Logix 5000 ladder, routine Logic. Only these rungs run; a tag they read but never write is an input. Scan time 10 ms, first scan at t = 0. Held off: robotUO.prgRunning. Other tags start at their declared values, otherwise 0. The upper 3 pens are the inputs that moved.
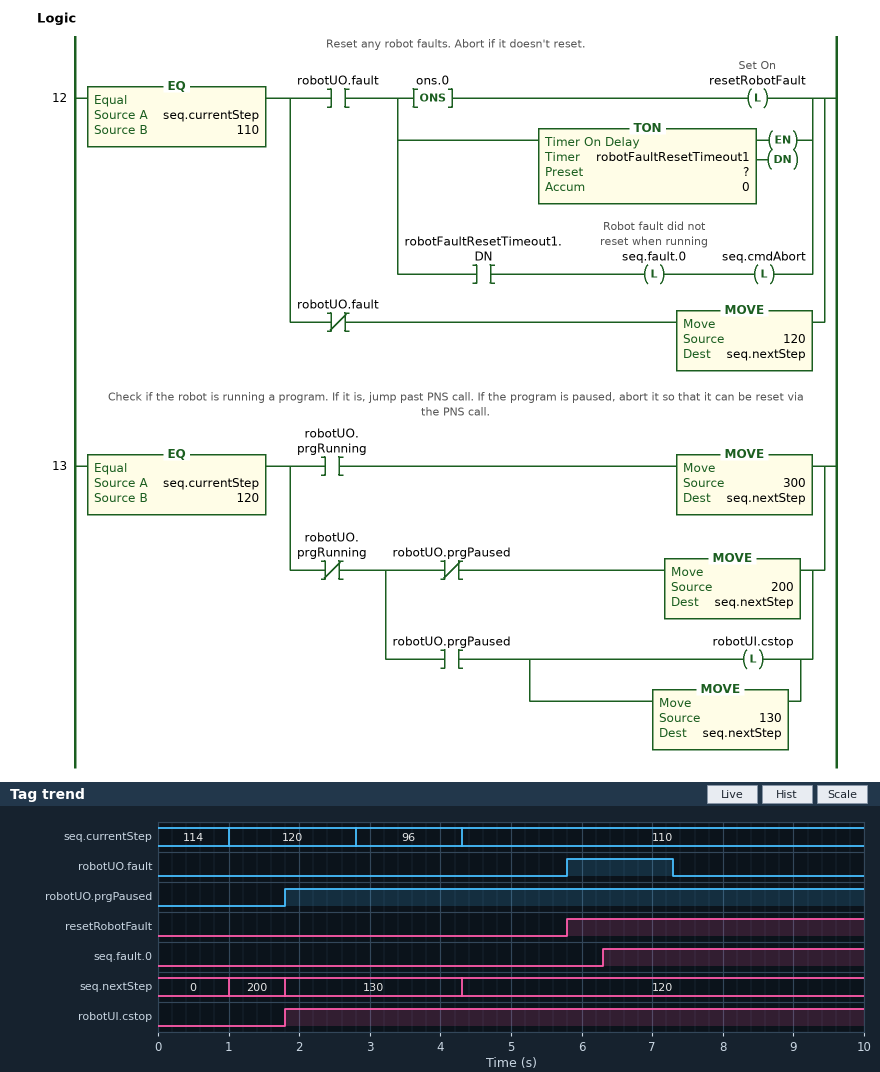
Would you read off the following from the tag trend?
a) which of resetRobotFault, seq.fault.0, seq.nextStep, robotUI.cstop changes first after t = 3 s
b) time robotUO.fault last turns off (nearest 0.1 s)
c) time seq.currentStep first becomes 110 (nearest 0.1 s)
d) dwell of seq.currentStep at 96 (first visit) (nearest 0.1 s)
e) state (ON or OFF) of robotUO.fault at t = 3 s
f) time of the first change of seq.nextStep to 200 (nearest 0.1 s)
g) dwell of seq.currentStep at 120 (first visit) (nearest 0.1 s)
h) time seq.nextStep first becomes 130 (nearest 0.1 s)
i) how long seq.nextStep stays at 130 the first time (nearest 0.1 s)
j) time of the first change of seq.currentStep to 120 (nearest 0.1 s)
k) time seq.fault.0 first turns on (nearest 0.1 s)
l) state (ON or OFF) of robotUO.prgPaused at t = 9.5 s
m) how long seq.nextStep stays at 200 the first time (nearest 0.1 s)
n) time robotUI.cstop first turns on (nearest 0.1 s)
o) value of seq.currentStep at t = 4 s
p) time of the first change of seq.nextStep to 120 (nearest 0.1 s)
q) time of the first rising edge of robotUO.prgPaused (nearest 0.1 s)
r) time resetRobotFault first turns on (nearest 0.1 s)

seq.nextStep
7.3 s
4.3 s
1.5 s
OFF
1.0 s
1.8 s
1.8 s
2.5 s
1.0 s
6.3 s
ON
0.8 s
1.8 s
96
4.3 s
1.8 s
5.8 s
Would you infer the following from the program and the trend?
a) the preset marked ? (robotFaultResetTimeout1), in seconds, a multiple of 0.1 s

0.5 s
